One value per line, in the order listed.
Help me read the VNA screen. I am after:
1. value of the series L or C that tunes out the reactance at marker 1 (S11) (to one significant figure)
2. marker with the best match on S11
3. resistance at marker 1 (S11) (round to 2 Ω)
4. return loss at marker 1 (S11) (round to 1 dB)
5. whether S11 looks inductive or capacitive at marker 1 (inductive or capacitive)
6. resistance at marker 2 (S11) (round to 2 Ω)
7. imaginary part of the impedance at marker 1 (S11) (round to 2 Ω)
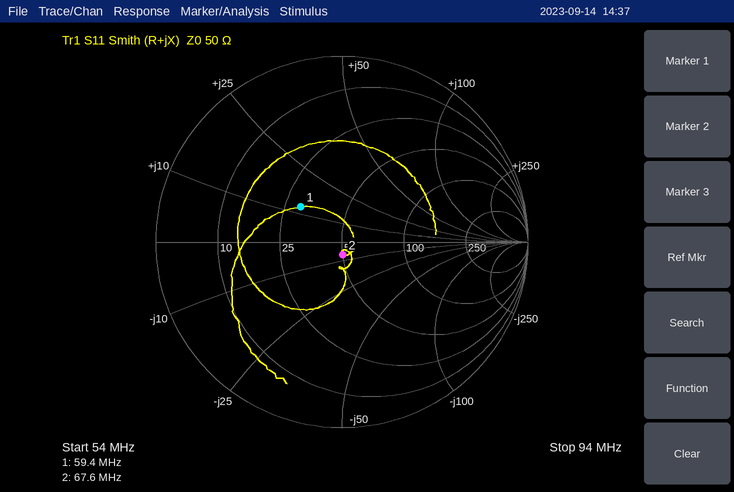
200 pF
marker 2
30 Ω
11 dB
inductive
50 Ω
+12 Ω
